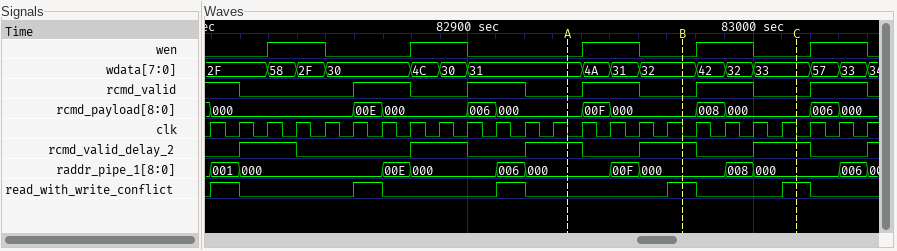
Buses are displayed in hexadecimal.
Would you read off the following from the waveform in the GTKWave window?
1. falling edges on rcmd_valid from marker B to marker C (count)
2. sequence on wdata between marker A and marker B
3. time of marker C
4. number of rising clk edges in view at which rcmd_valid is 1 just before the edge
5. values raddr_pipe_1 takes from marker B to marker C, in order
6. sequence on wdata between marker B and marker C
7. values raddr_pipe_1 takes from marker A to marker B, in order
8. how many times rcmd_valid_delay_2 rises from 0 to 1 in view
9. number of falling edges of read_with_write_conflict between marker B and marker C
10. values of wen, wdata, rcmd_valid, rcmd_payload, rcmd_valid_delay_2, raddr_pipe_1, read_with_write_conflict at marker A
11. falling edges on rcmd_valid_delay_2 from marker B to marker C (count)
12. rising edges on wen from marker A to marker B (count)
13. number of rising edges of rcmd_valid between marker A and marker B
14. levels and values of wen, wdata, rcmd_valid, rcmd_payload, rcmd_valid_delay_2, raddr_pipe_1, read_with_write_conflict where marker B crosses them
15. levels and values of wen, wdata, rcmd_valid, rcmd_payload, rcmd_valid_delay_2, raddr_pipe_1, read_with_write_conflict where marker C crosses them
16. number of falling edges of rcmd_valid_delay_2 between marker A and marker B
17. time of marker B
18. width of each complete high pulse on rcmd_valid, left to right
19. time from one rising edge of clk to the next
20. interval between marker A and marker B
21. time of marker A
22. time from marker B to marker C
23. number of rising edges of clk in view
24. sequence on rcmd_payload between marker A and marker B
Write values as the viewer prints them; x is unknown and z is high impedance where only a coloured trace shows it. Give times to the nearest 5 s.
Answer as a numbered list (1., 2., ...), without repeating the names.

1. 1
2. 31, 4A, 31, 32
3. 83015 s
4. 12
5. 000, 008, 000
6. 32, 42, 32, 33
7. 000, 00F, 000
8. 6
9. 1
10. wen=0, wdata=31, rcmd_valid=0, rcmd_payload=000, rcmd_valid_delay_2=1, raddr_pipe_1=000, read_with_write_conflict=0
11. 1
12. 1
13. 1
14. wen=0, wdata=32, rcmd_valid=0, rcmd_payload=000, rcmd_valid_delay_2=1, raddr_pipe_1=000, read_with_write_conflict=1
15. wen=0, wdata=33, rcmd_valid=0, rcmd_payload=000, rcmd_valid_delay_2=1, raddr_pipe_1=000, read_with_write_conflict=1
16. 1
17. 82975 s
18. 20 s, 20 s, 20 s, 20 s, 20 s
19. 10 s
20. 40 s
21. 82935 s
22. 40 s
23. 24
24. 000, 00F, 000
